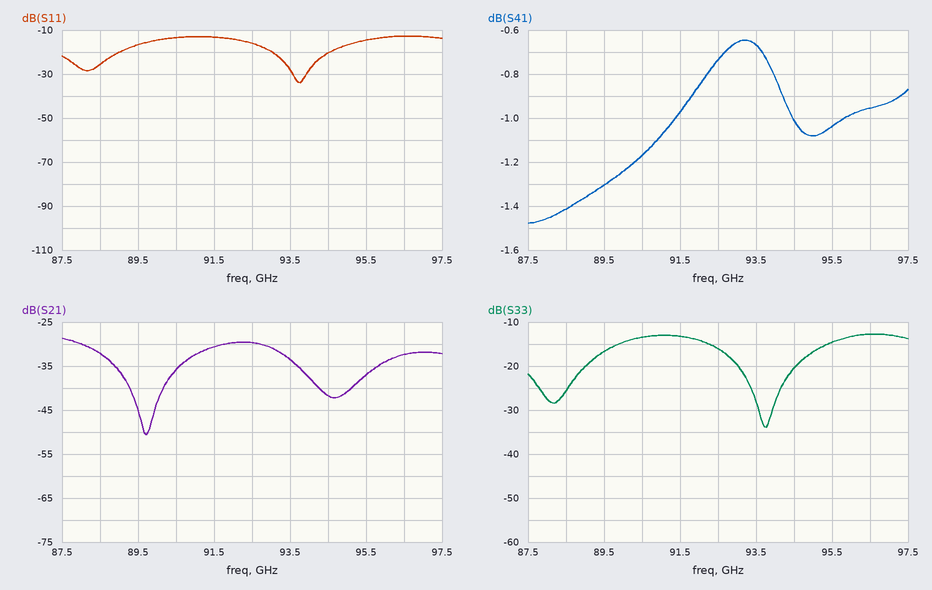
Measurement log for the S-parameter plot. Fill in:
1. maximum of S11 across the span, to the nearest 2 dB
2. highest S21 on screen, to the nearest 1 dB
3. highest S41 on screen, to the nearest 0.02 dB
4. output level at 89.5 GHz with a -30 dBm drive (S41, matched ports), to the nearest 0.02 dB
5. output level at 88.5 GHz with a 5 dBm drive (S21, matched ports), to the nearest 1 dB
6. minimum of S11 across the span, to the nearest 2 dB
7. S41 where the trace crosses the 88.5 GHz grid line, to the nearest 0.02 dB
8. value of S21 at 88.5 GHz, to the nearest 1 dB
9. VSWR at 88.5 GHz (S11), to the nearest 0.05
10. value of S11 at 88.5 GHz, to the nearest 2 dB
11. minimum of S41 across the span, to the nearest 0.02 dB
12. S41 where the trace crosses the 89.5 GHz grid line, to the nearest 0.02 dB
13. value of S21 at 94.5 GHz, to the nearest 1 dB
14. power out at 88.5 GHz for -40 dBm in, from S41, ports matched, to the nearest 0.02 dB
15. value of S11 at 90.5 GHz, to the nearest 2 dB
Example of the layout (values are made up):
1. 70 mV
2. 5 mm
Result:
1. -12 dB
2. -29 dB
3. -0.64 dB
4. -31.30 dBm
5. -27 dBm
6. -34 dB
7. -1.42 dB
8. -32 dB
9. 1.10
10. -26 dB
11. -1.48 dB
12. -1.30 dB
13. -42 dB
14. -41.42 dBm
15. -14 dB
